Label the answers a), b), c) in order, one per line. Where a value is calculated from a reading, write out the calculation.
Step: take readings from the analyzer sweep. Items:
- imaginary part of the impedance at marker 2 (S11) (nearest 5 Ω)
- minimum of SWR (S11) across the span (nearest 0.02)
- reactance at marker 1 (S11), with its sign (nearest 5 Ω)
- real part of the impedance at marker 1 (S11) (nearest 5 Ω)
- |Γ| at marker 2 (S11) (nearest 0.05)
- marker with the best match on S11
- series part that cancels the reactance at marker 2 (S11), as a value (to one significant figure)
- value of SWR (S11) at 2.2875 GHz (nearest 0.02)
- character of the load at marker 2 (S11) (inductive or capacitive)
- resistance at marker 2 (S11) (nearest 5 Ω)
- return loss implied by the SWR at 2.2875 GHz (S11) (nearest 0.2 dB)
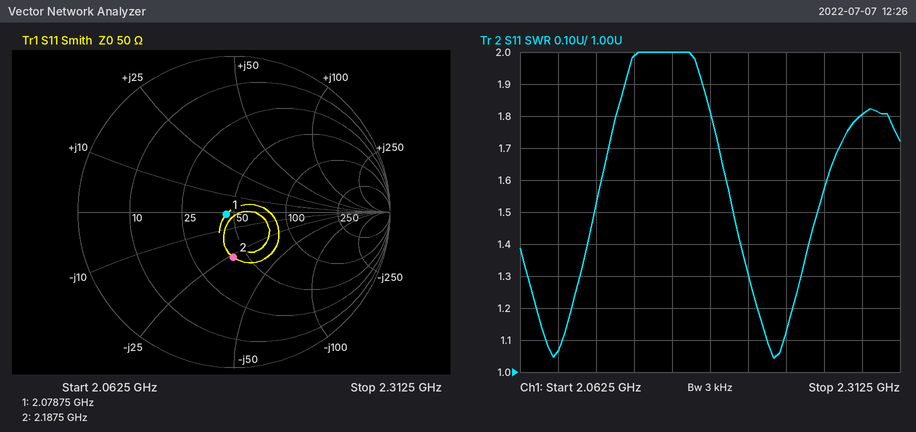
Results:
a) -25 Ω
b) 1.04
c) 0 Ω
d) 45 Ω
e) 0.30
f) marker 1
g) L = 25 Ω/(2π × 2.1875 GHz) ≈ 2 nH
h) 1.80
i) capacitive
j) 40 Ω
k) −20 log10((1.8 − 1)/(1.8 + 1)) ≈ 10.9 dB, so 10.8 dB to the nearest 0.2 dB
